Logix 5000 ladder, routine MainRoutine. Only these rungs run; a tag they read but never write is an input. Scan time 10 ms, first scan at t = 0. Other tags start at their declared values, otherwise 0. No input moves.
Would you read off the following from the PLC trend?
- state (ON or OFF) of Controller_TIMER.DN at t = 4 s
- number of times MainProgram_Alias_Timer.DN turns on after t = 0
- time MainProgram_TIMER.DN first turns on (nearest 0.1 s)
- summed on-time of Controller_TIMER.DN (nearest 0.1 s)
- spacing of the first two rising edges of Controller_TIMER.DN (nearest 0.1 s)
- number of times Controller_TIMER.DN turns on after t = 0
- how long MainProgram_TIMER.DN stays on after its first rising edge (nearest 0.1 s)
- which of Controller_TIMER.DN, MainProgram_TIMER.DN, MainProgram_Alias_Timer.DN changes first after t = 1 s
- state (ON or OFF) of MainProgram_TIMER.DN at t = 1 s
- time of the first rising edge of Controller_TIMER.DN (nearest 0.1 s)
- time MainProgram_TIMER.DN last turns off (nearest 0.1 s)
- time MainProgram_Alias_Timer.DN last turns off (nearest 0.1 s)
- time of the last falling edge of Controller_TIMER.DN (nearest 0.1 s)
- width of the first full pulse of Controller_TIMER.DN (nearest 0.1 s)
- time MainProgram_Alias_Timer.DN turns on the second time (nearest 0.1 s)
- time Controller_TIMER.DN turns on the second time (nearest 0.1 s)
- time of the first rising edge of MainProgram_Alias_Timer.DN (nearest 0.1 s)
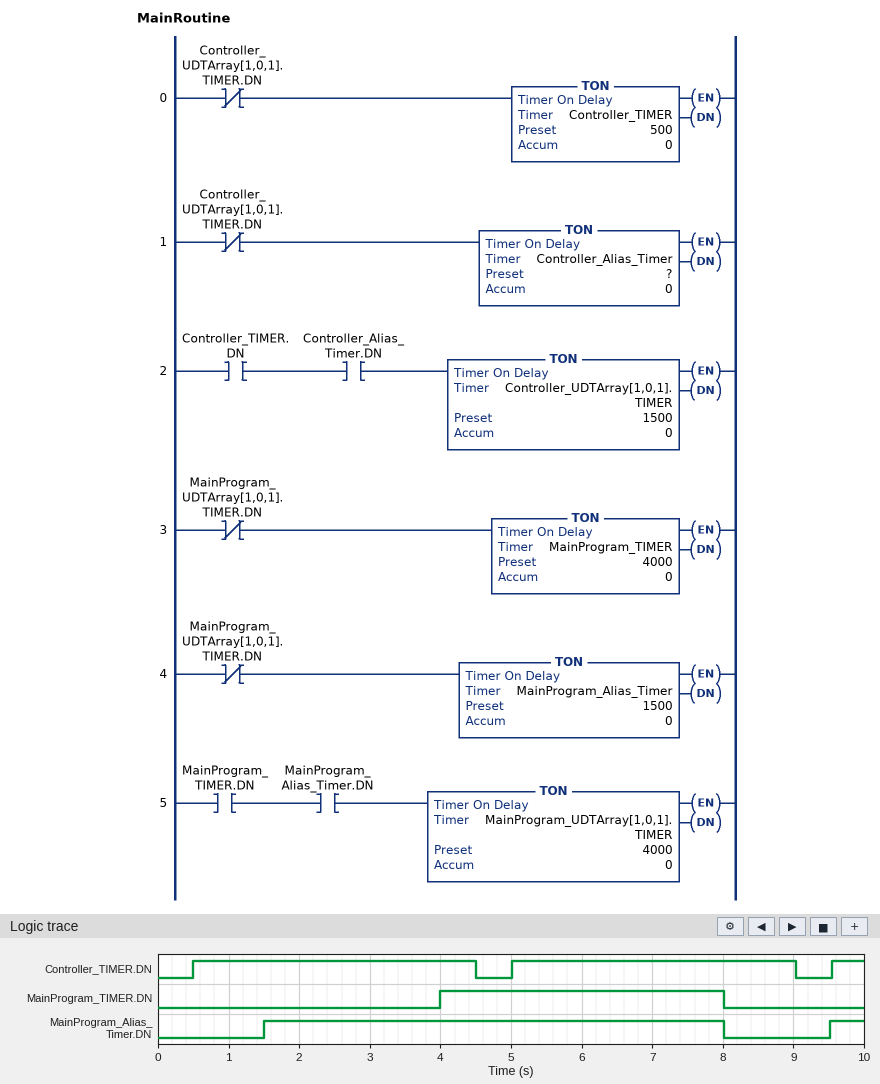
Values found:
ON
2
4.0 s
8.5 s
4.5 s
3
4.0 s
MainProgram_Alias_Timer.DN
OFF
0.5 s
8.0 s
8.0 s
9.0 s
4.0 s
9.5 s
5.0 s
1.5 s
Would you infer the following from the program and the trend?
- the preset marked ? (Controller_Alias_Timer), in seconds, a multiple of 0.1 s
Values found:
3.0 s
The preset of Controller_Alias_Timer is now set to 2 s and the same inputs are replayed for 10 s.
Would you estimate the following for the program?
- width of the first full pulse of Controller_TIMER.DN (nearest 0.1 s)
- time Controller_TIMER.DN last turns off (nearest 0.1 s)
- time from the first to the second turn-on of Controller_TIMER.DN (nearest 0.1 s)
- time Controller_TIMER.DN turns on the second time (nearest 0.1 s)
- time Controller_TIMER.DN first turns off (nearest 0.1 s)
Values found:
3.0 s
7.0 s
3.5 s
4.0 s
3.5 s
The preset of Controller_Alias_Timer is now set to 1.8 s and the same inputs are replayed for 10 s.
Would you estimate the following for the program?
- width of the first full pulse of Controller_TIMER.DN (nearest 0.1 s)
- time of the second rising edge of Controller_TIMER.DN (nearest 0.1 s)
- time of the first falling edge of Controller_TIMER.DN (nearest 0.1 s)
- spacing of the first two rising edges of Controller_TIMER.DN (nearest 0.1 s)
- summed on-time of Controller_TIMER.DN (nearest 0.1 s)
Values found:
2.8 s
3.8 s
3.3 s
3.3 s
8.4 s
